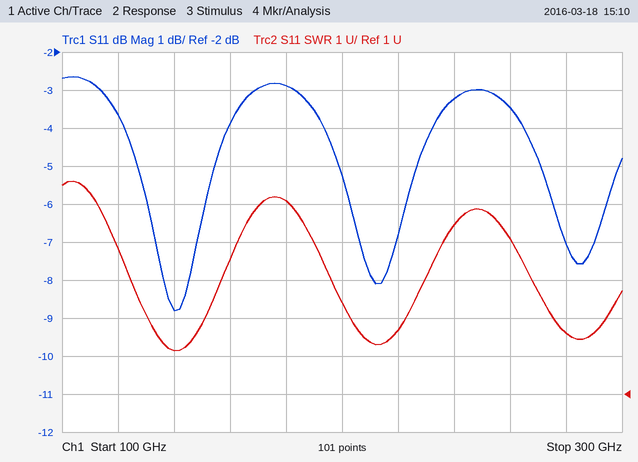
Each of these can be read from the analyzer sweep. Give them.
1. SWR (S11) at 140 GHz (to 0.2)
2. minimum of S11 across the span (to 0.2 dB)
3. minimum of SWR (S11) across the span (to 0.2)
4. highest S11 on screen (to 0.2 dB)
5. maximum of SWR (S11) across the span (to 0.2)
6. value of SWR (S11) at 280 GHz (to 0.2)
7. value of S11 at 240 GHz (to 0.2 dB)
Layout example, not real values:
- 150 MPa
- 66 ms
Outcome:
- 2.2
- -8.8 dB
- 2.2
- -2.6 dB
- 6.6
- 2.6
- -3.2 dB
